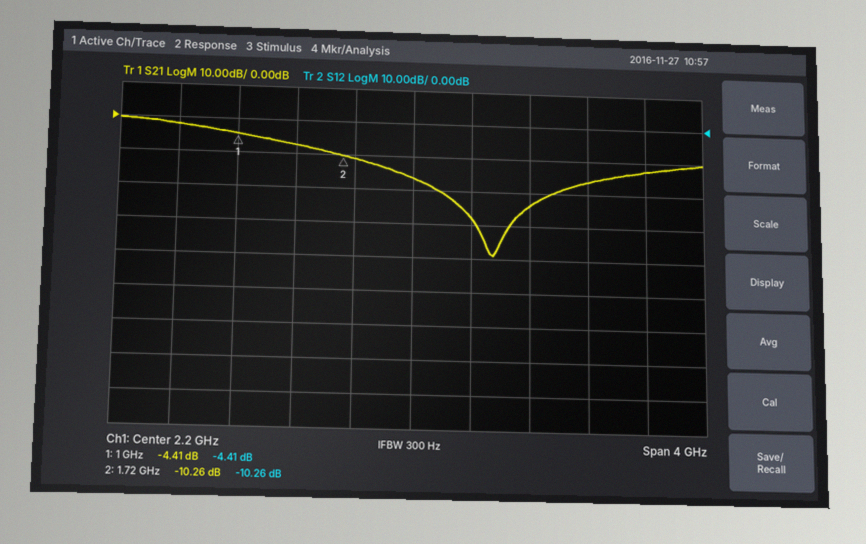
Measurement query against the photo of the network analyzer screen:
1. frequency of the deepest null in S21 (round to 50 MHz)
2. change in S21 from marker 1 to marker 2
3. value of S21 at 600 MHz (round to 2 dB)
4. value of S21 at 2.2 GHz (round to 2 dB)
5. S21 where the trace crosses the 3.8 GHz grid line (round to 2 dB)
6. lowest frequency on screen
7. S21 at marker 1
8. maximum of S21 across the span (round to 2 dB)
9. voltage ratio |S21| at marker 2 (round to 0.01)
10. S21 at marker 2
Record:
2.75 GHz
-5.85 dB
-2 dB
-16 dB
-12 dB
200 MHz
-4.41 dB
0 dB
0.31
-10.26 dB
